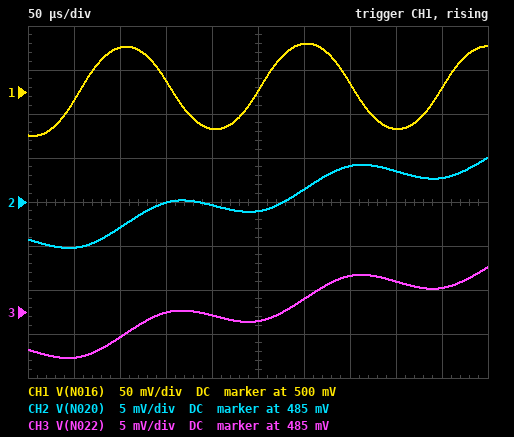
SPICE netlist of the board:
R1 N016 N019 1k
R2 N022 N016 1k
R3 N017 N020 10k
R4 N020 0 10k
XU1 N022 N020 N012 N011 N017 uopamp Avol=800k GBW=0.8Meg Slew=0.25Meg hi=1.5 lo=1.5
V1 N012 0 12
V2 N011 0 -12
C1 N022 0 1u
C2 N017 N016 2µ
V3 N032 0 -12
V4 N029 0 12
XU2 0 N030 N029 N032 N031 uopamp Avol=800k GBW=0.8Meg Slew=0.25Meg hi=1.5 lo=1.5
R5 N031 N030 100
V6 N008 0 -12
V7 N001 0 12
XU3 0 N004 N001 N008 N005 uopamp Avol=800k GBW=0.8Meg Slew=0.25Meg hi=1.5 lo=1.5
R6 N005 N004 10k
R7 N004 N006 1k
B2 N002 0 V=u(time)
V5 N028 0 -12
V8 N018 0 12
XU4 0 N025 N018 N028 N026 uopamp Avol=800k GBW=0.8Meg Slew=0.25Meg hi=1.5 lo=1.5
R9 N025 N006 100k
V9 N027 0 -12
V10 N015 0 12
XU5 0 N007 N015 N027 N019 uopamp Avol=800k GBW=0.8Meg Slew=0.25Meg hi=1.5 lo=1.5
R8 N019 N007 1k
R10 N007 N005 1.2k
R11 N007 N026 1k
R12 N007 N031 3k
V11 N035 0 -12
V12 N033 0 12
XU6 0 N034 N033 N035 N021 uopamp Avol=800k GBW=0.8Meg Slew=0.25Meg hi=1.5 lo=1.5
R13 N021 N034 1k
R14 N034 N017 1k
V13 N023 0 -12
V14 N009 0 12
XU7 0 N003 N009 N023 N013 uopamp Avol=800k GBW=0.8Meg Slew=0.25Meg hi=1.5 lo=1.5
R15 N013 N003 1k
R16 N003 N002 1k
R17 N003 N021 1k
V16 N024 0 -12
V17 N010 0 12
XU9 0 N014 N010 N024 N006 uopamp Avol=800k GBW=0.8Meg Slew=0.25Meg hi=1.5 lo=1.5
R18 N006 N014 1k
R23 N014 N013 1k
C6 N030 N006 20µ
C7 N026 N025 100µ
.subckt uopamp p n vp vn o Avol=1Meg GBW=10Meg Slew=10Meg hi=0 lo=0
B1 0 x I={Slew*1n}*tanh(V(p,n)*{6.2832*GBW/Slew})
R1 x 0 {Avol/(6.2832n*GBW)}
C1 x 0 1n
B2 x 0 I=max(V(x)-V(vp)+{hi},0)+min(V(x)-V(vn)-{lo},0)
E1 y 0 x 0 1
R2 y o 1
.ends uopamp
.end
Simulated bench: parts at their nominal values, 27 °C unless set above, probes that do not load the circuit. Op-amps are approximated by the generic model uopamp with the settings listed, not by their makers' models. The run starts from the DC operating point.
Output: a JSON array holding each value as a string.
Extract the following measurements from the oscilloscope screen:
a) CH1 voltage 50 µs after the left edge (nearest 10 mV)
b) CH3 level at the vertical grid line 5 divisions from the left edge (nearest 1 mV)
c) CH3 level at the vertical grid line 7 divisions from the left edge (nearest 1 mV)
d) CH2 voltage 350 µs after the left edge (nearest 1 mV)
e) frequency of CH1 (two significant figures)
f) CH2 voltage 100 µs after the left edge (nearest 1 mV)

["490 mV", "484 mV", "489 mV", "489 mV", "5.1 kHz", "482 mV"]
